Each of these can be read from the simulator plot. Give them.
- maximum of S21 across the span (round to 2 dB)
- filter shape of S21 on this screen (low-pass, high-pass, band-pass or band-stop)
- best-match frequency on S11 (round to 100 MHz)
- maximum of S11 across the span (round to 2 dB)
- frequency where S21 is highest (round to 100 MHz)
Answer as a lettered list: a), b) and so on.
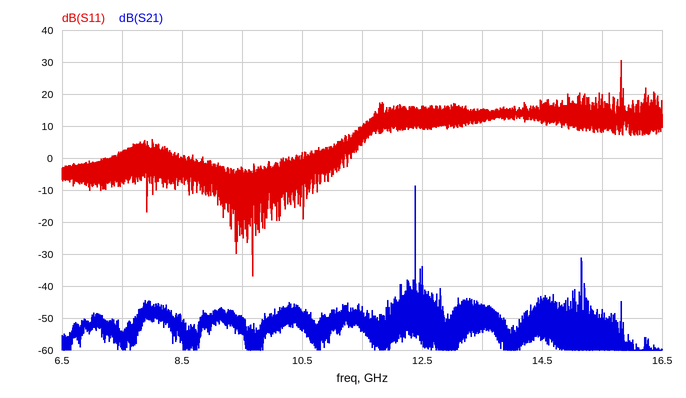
a) -8 dB
b) band-pass
c) 9.7 GHz
d) 30 dB
e) 12.4 GHz
